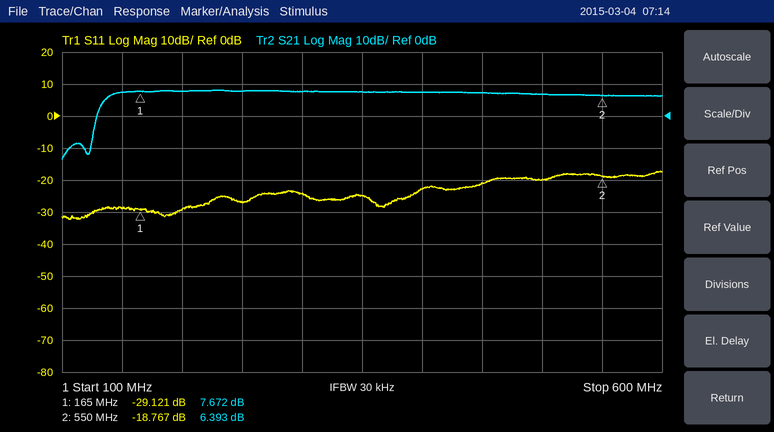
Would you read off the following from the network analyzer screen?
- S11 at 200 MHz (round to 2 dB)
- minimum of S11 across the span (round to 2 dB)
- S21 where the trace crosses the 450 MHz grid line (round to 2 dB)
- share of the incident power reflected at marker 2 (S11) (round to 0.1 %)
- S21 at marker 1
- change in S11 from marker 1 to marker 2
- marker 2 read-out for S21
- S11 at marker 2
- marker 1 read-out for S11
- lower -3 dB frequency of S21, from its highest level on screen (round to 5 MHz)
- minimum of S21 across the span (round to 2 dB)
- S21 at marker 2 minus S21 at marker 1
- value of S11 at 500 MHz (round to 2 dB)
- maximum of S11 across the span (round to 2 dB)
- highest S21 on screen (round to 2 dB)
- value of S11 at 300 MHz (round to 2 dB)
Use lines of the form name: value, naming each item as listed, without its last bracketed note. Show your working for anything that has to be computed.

S11 at 200 MHz: -30 dB
minimum of S11 across the span: -32 dB
S21 where the trace crosses the 450 MHz grid line: 8 dB
share of the incident power reflected at marker 2 (S11): 10^(-18.767/10) ≈ 1.3 %
S21 at marker 1: 7.672 dB
change in S11 from marker 1 to marker 2: -18.767 − (-29.121) = 10.354 dB
marker 2 read-out for S21: 6.393 dB
S11 at marker 2: -18.767 dB
marker 1 read-out for S11: -29.121 dB
lower -3 dB frequency of S21, from its highest level on screen: 135 MHz
minimum of S21 across the span: -14 dB
S21 at marker 2 minus S21 at marker 1: 6.393 − (7.672) = -1.279 dB
value of S11 at 500 MHz: -20 dB
maximum of S11 across the span: -18 dB
highest S21 on screen: 8 dB
value of S11 at 300 MHz: -24 dB
